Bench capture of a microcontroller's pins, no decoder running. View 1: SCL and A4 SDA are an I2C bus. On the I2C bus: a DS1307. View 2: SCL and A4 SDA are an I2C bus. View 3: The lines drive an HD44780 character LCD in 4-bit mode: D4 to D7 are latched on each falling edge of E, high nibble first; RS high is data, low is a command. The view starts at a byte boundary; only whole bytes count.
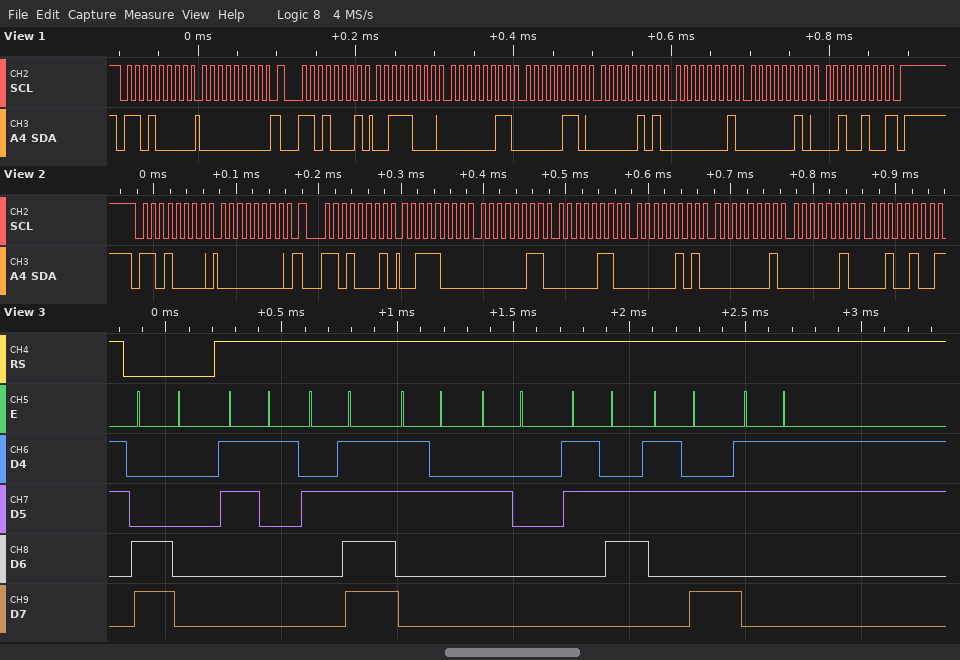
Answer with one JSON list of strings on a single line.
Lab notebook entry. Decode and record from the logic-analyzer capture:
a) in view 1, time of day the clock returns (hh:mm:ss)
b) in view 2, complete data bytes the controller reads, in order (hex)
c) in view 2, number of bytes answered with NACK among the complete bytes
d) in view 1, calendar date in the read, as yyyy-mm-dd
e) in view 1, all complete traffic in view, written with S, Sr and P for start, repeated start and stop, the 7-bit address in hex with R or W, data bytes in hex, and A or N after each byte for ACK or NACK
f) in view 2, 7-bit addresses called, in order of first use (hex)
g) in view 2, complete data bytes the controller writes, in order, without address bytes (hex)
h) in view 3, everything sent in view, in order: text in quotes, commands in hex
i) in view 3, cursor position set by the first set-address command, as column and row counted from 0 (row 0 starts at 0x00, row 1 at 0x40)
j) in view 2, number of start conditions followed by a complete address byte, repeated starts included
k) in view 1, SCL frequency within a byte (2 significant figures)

["06:03:38", "38 03 06 05 01 02 24", "1", "2024-02-01", "S 68W A 00 A Sr 68R A 38 A 03 A 06 A 05 A 01 A 02 A 24 N P", "0x68", "00", "0xC0 \"1/2 6:3\"", "column 0, row 1", "2", "100 kHz"]
